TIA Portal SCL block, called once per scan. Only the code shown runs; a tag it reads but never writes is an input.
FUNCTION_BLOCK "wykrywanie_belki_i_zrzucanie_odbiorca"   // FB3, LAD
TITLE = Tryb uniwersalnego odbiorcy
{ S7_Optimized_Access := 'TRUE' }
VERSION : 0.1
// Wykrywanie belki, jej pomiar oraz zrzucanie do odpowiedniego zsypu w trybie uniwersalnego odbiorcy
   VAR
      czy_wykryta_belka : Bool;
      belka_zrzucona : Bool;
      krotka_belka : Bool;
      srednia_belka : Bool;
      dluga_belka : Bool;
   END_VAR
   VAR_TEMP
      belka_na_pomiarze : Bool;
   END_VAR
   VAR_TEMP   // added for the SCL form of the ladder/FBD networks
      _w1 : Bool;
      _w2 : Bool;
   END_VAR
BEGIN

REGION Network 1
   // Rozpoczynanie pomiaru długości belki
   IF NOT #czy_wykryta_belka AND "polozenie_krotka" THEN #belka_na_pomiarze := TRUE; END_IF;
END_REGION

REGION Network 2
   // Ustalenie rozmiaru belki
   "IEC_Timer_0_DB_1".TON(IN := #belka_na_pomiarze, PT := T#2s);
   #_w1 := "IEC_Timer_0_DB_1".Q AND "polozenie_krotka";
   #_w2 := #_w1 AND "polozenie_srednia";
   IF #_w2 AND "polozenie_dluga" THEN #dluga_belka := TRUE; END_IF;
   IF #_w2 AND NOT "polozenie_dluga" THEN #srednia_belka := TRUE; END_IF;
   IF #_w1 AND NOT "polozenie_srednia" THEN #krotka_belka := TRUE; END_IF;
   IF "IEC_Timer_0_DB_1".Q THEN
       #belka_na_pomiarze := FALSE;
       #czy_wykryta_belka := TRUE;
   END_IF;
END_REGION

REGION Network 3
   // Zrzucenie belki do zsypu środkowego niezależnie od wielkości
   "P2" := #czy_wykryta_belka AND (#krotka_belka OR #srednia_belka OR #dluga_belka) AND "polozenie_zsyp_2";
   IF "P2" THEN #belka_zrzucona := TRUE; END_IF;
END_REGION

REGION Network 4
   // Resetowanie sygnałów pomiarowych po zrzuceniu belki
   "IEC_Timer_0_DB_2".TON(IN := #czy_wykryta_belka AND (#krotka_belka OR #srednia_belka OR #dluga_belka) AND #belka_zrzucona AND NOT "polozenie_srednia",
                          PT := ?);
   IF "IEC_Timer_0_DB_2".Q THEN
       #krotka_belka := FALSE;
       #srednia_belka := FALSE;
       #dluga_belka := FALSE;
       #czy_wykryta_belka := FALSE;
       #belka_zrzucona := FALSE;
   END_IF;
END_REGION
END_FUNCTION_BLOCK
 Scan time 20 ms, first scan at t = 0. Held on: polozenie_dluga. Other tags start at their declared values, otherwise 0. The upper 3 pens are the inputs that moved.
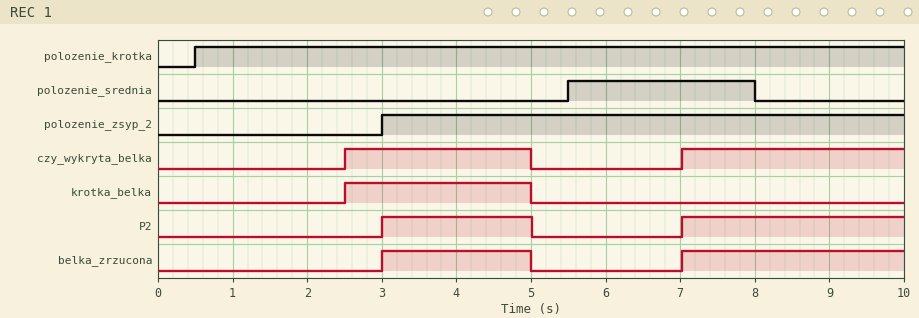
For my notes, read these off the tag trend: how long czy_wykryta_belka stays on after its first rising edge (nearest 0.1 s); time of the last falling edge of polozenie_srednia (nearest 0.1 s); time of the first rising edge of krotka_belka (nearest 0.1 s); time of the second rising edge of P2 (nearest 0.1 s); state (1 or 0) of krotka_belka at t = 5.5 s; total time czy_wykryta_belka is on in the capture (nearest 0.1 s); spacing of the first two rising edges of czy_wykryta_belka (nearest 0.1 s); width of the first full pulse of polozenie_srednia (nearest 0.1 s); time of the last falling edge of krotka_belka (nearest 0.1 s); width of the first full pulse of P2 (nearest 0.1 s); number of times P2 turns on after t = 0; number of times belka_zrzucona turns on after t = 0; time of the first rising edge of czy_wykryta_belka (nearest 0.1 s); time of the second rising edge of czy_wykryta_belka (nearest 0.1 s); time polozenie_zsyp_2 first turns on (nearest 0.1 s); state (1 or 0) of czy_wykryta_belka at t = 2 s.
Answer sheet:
2.5 s
8.0 s
2.5 s
7.0 s
0
5.5 s
4.5 s
2.5 s
5.0 s
2.0 s
2
2
2.5 s
7.0 s
3.0 s
0
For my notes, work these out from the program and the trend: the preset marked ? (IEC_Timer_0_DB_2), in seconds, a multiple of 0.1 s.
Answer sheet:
2.0 s
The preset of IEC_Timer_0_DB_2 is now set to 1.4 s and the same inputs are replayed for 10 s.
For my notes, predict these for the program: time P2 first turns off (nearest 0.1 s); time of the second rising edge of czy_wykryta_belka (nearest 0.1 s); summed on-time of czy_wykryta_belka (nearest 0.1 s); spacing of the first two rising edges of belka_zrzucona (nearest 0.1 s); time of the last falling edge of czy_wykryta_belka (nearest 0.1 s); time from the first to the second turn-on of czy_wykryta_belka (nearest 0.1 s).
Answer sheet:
4.4 s
6.4 s
4.9 s
3.4 s
9.4 s
3.9 s
